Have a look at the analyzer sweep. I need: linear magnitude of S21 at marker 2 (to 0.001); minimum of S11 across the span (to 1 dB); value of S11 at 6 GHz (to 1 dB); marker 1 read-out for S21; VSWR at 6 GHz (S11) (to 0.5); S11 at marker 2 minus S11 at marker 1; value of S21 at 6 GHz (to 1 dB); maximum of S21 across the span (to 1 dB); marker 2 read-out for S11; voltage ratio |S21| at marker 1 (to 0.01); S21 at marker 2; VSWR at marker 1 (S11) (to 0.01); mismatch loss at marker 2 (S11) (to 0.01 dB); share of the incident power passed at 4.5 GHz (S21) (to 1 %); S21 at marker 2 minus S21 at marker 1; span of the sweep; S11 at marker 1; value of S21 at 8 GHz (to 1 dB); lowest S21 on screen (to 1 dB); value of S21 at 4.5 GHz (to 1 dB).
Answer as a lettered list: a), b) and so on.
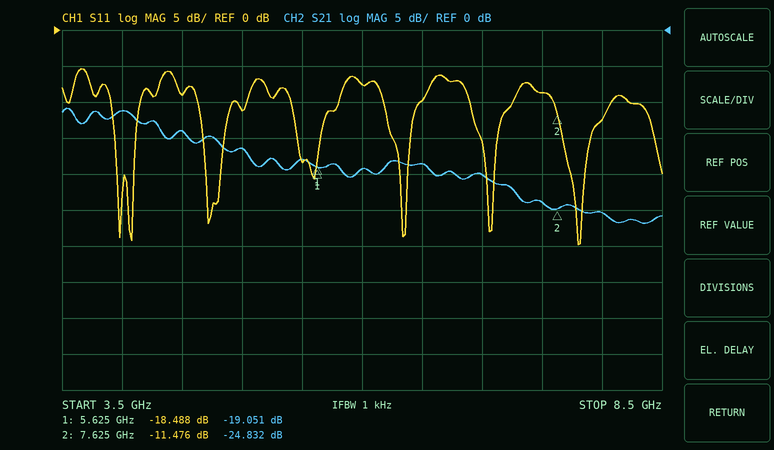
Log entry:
a) 0.057
b) -30 dB
c) -8 dB
d) -19.051 dB
e) 2.5
f) 7.012 dB
g) -19 dB
h) -11 dB
i) -11.476 dB
j) 0.11
k) -24.832 dB
l) 1.27
m) 0.32 dB
n) 4 %
o) -5.781 dB
p) 5 GHz
q) -18.488 dB
r) -25 dB
s) -27 dB
t) -14 dB
